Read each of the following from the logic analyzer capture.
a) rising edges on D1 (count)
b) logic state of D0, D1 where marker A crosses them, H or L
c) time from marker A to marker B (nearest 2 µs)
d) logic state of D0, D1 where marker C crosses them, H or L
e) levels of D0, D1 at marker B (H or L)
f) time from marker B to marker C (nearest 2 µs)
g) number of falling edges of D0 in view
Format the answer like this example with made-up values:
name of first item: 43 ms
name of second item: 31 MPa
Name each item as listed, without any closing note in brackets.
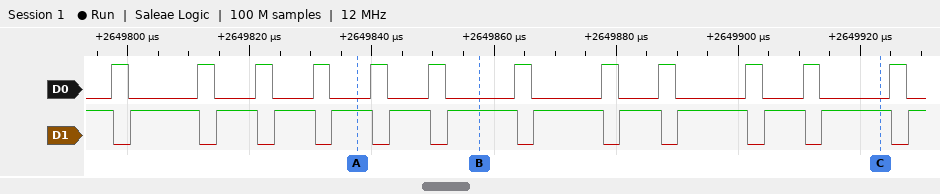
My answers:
rising edges on D1: 12
logic state of D0, D1 where marker A crosses them, H or L: D0=L, D1=H
time from marker A to marker B: 20 µs
logic state of D0, D1 where marker C crosses them, H or L: D0=L, D1=H
levels of D0, D1 at marker B: D0=L, D1=H
time from marker B to marker C: 66 µs
number of falling edges of D0 in view: 12
